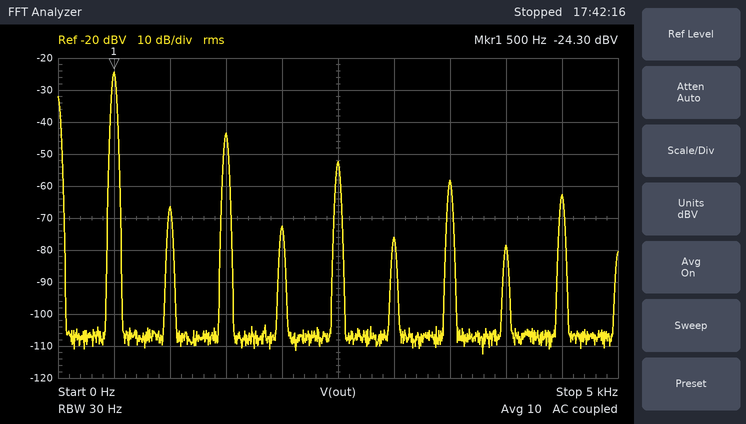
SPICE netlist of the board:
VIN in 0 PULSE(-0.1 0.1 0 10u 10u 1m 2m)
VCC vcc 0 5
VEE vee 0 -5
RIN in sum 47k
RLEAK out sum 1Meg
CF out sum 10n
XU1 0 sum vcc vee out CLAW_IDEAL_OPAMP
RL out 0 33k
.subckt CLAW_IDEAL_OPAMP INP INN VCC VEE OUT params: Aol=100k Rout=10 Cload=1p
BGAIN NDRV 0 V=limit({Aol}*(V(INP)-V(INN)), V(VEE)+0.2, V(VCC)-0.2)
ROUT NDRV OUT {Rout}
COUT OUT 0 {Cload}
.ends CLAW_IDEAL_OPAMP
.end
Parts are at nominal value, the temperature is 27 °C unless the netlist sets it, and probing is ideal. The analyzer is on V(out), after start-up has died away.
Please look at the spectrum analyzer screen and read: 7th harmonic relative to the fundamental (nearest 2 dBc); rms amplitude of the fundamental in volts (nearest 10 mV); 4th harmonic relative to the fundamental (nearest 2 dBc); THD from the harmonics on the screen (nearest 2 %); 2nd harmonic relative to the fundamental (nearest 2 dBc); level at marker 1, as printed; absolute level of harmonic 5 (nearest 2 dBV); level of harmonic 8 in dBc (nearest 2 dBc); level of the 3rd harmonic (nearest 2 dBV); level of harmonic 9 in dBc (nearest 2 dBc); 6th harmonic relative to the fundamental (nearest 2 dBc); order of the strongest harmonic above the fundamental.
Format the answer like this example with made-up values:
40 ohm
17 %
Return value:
-34 dBc
60 mV
-48 dBc
12 %
-42 dBc
-24.30 dBV
-52 dBV
-54 dBc
-44 dBV
-38 dBc
-52 dBc
3
